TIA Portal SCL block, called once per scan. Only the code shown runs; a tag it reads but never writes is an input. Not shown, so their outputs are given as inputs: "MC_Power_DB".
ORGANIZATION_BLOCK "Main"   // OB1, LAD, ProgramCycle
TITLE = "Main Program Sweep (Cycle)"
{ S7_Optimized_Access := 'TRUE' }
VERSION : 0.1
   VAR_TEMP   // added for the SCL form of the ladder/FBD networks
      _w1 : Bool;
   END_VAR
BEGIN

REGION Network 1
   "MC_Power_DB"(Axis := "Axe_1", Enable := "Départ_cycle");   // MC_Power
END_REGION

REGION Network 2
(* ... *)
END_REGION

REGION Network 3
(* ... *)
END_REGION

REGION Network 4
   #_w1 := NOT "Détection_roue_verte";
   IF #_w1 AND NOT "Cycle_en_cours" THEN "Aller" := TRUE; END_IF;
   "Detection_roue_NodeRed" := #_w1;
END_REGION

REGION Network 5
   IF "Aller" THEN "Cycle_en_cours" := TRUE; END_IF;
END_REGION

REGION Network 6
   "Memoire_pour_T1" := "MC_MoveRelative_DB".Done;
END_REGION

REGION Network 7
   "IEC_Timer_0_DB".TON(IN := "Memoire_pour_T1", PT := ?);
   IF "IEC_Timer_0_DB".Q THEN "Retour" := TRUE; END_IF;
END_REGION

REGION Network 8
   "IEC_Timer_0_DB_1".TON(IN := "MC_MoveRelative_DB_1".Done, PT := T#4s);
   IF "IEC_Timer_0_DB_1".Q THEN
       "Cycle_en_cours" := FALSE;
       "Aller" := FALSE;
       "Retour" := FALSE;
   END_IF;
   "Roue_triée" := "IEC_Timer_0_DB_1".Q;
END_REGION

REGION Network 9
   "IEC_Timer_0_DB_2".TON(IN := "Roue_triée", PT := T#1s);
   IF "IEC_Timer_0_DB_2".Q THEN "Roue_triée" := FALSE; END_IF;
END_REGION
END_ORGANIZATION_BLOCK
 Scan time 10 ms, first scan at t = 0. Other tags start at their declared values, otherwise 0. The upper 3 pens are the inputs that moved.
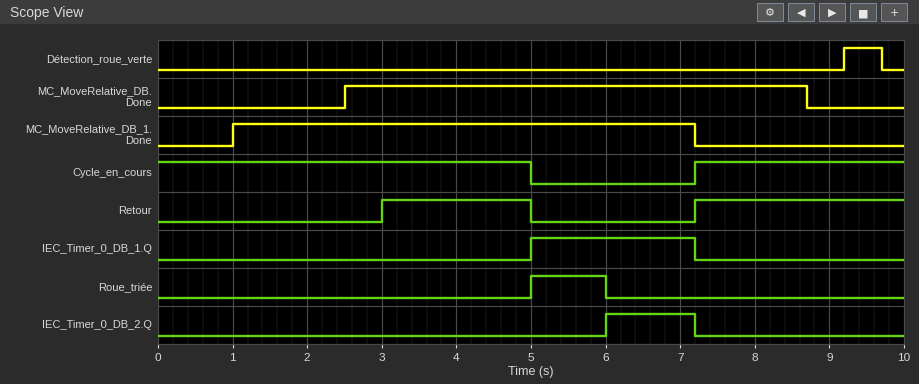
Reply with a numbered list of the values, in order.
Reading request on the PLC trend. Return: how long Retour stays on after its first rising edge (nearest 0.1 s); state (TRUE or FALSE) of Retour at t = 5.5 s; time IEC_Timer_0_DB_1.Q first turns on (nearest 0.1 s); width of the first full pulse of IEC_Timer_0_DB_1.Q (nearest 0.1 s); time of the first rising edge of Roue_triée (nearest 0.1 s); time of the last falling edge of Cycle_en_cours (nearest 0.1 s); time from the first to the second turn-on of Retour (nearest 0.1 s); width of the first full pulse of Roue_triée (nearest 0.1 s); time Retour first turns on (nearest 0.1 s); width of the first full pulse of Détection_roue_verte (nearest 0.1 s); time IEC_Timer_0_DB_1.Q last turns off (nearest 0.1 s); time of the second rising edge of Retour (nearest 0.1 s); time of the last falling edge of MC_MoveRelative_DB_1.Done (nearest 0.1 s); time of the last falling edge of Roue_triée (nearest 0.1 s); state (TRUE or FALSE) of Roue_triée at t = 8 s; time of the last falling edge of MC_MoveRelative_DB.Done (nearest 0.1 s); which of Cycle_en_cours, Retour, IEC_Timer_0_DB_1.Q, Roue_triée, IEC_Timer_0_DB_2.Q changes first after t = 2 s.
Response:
1. 2.0 s
2. FALSE
3. 5.0 s
4. 2.2 s
5. 5.0 s
6. 5.0 s
7. 4.2 s
8. 1.0 s
9. 3.0 s
10. 0.5 s
11. 7.2 s
12. 7.2 s
13. 7.2 s
14. 6.0 s
15. FALSE
16. 8.7 s
17. Retour
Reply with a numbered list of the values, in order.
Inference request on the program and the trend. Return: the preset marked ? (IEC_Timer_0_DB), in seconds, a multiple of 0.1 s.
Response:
1. 0.5 s
